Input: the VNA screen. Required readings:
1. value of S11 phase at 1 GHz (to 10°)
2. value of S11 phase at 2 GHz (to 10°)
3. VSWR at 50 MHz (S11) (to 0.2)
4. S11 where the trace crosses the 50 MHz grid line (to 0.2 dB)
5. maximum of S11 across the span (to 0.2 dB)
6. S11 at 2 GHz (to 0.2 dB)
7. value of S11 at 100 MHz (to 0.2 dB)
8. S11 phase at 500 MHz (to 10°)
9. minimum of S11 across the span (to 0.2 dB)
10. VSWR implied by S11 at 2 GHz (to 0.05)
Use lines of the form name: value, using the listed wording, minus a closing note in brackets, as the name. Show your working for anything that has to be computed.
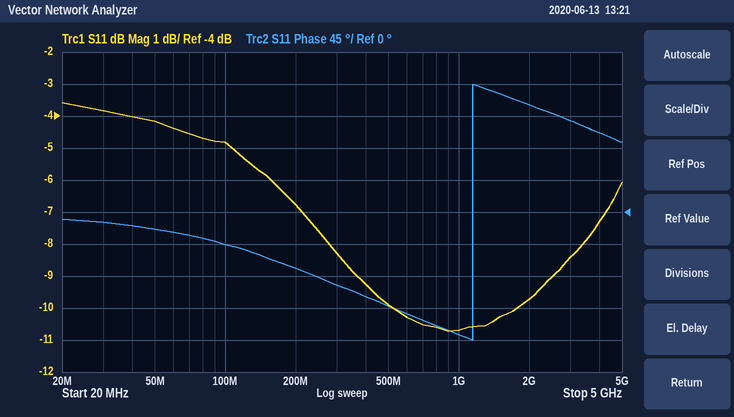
value of S11 phase at 1 GHz: -170°
value of S11 phase at 2 GHz: 150°
VSWR at 50 MHz (S11): |Γ| = 10^(-4.2/20) = 0.6166; VSWR = (1 + 0.6166)/(1 − 0.6166) ≈ 4.2
S11 where the trace crosses the 50 MHz grid line: -4.2 dB
maximum of S11 across the span: -3.6 dB
S11 at 2 GHz: -9.8 dB
value of S11 at 100 MHz: -4.8 dB
S11 phase at 500 MHz: -130°
minimum of S11 across the span: -10.8 dB
VSWR implied by S11 at 2 GHz: |Γ| = 10^(-9.8/20) = 0.3236; VSWR = (1 + 0.3236)/(1 − 0.3236) ≈ 1.96, so 1.95 to the nearest 0.05
